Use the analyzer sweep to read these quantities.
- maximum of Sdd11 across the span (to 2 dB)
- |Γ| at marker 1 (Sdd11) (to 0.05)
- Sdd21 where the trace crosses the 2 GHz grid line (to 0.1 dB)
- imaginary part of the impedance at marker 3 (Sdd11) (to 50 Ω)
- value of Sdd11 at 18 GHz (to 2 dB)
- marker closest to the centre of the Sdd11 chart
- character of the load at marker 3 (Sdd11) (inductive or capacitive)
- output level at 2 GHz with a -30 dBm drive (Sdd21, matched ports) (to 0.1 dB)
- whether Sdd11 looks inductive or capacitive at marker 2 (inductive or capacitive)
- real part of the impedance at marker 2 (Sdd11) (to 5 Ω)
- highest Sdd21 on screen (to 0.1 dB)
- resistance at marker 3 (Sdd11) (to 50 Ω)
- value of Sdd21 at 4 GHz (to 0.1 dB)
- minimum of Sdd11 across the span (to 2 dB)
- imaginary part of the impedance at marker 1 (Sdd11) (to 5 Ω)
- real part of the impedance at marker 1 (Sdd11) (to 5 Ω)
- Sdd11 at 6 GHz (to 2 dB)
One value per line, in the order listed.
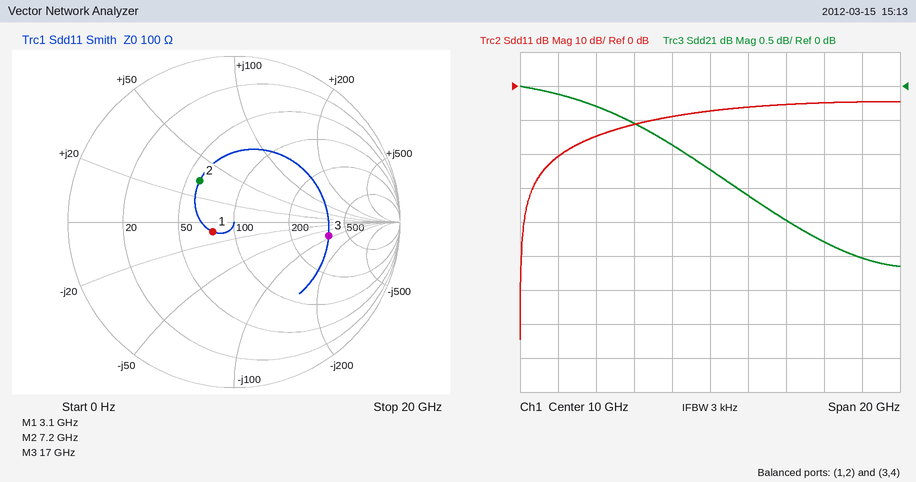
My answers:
-4 dB
0.15
-0.1 dB
-100 Ω
-4 dB
marker 1
capacitive
-30.1 dBm
inductive
60 Ω
0.0 dB
350 Ω
-0.3 dB
-74 dB
-10 Ω
75 Ω
-12 dB
